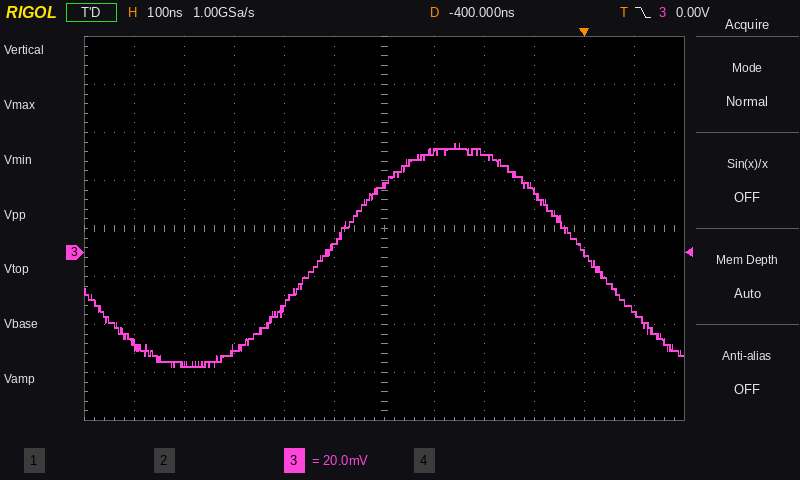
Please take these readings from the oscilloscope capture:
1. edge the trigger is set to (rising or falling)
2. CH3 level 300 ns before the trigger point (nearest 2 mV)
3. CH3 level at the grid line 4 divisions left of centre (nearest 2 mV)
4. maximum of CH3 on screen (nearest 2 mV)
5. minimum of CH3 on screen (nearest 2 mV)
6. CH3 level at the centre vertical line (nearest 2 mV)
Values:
falling
42 mV
-46 mV
46 mV
-48 mV
28 mV
